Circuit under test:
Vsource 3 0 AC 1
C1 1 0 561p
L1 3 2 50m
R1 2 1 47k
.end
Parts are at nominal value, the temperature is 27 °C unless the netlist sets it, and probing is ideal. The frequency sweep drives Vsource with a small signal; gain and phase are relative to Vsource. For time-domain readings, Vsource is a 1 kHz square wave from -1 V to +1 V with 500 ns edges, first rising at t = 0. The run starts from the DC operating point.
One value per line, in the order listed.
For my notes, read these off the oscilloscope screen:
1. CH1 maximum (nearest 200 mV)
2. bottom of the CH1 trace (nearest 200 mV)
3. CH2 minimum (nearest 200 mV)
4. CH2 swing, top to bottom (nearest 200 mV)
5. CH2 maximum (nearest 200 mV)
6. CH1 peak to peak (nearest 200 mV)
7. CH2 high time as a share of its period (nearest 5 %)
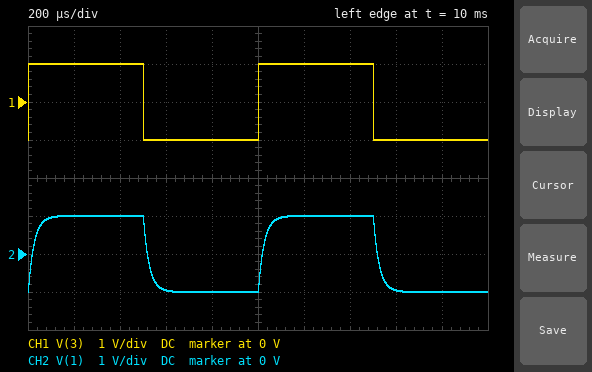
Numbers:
1.0 V
-1.0 V
-1.0 V
2.0 V
1.0 V
2.0 V
50 %
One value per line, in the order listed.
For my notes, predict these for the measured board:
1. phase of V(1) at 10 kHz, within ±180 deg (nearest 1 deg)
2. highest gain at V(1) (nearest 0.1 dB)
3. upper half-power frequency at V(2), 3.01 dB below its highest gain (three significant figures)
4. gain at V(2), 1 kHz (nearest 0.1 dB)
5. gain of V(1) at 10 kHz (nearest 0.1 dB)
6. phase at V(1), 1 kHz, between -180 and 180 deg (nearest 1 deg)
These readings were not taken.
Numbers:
-62 deg
0 dB
147 kHz
0 dB
-5.5 dB
-9 deg
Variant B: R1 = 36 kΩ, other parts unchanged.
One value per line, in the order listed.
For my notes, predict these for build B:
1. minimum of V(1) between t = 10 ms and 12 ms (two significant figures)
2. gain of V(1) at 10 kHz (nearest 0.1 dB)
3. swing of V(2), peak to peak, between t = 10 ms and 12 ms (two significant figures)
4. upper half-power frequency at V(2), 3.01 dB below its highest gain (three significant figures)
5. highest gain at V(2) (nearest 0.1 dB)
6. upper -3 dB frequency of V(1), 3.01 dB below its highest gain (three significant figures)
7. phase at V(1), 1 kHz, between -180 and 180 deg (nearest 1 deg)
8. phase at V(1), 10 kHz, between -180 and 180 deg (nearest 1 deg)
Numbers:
-1.0 V
-3.8 dB
2.2 V
112 kHz
0.4 dB
8.46 kHz
-7 deg
-55 deg
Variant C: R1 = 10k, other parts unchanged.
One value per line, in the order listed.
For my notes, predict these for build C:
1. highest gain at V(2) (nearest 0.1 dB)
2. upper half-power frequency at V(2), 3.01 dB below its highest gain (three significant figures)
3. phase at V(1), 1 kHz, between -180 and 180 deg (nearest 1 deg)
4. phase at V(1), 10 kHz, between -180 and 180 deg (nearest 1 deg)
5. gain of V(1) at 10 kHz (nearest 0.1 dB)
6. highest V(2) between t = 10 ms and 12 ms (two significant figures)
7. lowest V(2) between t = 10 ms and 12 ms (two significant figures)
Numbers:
3.1 dB
42.2 kHz
-2 deg
-22 deg
0.4 dB
1.6 V
-1.6 V
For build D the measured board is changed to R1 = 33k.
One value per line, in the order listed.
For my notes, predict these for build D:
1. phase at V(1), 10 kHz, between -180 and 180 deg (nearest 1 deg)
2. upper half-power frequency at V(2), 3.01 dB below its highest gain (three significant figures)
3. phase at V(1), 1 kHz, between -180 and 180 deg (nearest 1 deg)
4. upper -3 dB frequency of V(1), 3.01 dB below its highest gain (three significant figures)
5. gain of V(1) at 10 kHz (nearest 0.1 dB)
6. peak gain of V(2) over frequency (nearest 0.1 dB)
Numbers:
-53 deg
102 kHz
-7 deg
9.36 kHz
-3.3 dB
0.5 dB
